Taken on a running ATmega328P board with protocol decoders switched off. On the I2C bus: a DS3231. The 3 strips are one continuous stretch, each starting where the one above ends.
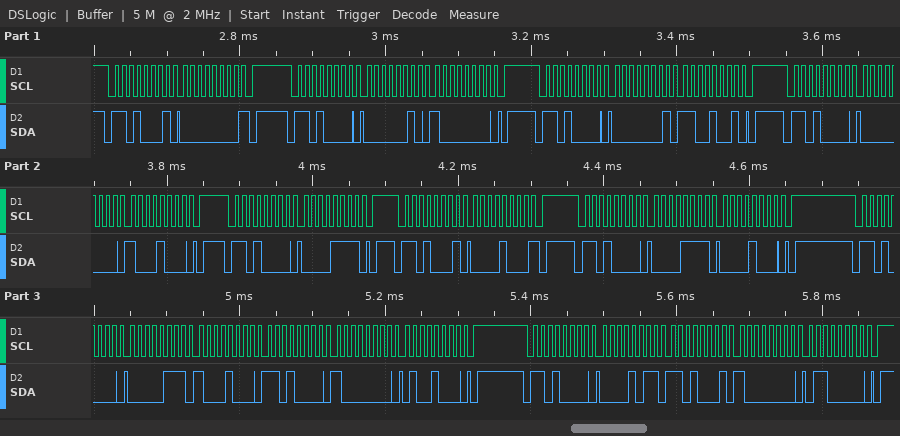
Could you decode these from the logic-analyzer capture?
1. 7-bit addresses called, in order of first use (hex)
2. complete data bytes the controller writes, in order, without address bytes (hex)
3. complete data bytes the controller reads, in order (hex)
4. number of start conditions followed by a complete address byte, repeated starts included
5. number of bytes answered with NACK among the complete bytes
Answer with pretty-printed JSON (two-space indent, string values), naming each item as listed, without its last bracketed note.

{
  "7-bit addresses called, in order of first use": "0x68",
  "complete data bytes the controller writes, in order, without address bytes": "02 80 01 C9 00 88 0F 0F 08 07 88 D0 80 48 0B D1 80 60",
  "complete data bytes the controller reads, in order": "00 08",
  "number of start conditions followed by a complete address byte, repeated starts included": "9",
  "number of bytes answered with NACK among the complete bytes": "2"
}
